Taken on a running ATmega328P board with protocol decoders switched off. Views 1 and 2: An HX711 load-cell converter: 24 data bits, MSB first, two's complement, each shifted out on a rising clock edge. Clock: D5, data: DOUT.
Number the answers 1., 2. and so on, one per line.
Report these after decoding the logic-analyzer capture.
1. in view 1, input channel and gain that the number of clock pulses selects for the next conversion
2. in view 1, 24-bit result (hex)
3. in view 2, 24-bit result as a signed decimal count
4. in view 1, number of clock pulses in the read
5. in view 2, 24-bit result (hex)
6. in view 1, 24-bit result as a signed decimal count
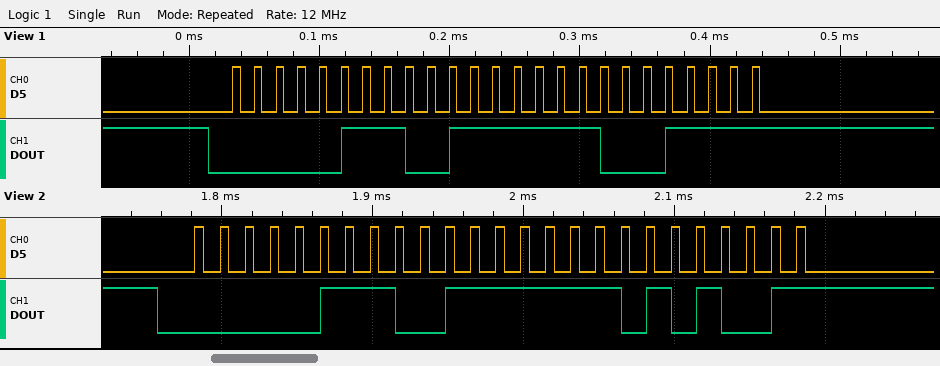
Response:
1. channel A, gain 128
2. 0x073F8F
3. 475049
4. 25
5. 0x073FA9
6. 475023
